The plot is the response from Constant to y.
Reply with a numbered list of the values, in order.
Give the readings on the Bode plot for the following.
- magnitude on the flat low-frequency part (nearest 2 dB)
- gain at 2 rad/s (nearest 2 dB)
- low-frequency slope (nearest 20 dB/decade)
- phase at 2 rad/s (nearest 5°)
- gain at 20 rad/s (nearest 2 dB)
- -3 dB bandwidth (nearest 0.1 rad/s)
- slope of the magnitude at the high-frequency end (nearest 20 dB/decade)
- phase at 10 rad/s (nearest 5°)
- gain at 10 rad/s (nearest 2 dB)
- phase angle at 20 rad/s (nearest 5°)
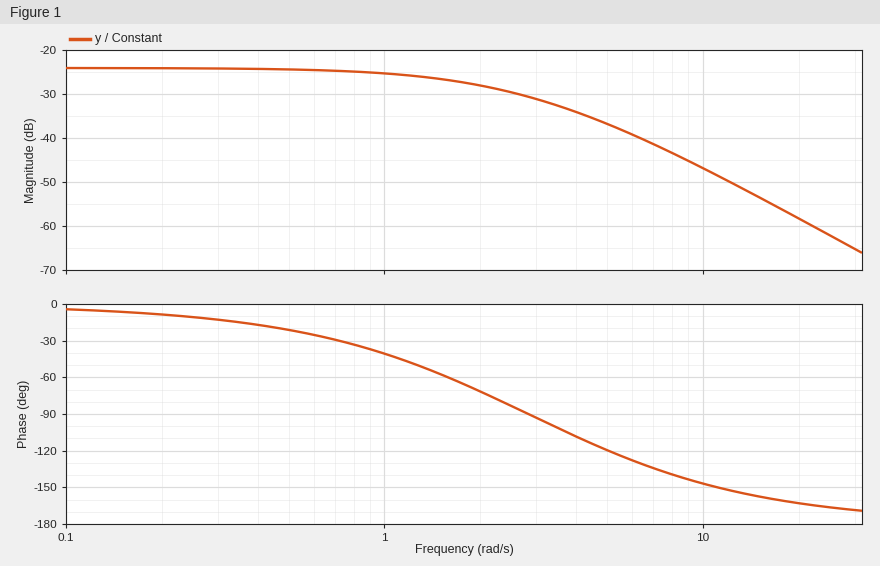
1. -24 dB
2. -28 dB
3. 0 dB/decade
4. -70°
5. -58 dB
6. 1.7 rad/s
7. -40 dB/decade
8. -145°
9. -46 dB
10. -165°
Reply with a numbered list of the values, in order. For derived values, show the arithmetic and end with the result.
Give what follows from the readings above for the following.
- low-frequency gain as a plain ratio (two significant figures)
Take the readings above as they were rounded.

1. 10^(-24 / 20) = 0.063
